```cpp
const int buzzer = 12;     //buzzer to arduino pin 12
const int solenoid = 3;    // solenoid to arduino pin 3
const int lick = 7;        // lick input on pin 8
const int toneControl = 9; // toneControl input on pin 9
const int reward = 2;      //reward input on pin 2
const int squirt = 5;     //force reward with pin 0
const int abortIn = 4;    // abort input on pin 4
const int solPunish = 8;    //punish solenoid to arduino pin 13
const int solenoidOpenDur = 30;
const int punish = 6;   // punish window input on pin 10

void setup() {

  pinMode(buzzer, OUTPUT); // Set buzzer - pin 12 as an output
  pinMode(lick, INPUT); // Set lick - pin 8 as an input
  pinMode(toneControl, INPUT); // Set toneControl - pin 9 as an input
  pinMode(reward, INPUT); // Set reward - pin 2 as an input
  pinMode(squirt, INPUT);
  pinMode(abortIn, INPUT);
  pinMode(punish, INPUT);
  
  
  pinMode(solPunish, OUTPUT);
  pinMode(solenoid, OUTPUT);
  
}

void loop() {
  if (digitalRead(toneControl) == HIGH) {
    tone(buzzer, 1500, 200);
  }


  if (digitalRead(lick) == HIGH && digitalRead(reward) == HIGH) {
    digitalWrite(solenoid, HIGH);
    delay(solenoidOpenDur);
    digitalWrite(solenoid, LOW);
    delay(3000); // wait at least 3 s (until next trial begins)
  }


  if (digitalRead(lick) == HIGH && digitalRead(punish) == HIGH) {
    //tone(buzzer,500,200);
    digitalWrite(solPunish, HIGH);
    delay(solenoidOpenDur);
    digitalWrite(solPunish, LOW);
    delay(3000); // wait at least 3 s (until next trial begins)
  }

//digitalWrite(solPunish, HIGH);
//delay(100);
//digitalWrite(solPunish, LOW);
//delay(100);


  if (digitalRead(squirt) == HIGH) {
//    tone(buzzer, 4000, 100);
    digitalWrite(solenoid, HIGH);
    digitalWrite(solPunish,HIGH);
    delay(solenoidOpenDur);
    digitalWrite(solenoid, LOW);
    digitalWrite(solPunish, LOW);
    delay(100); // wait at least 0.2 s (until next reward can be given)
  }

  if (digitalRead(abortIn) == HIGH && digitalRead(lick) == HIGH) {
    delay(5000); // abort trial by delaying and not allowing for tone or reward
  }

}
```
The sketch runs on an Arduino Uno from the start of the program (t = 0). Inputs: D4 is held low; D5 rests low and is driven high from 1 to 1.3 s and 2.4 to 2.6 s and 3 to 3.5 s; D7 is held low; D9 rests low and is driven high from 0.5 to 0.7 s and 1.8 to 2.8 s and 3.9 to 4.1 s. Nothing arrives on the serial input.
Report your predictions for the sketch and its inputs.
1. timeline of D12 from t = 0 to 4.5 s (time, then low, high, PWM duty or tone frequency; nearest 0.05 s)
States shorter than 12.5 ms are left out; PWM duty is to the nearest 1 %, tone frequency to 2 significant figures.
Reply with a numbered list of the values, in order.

1. 0 s low; 0.5 s tone 1500 Hz; 0.9 s low; 1.8 s tone 1500 Hz; 3 s low; 3.9 s tone 1500 Hz; 4.3 s low
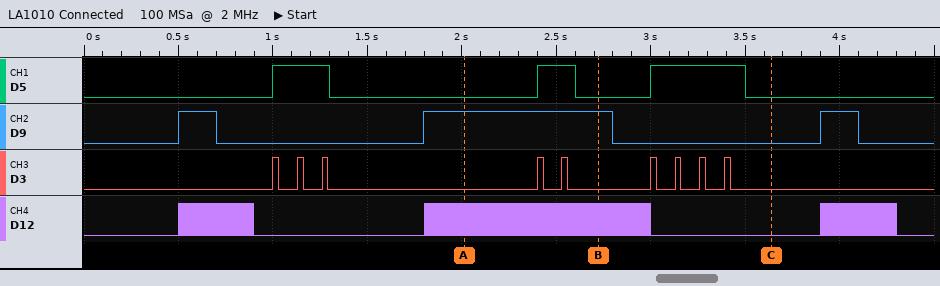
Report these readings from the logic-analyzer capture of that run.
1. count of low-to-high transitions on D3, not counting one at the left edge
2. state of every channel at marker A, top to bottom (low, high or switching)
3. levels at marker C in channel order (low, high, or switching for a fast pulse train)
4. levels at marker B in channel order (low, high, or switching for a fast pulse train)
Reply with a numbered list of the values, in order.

1. 9
2. D5 low, D9 high, D3 low, D12 switching
3. D5 low, D9 low, D3 low, D12 low
4. D5 low, D9 high, D3 low, D12 switching
